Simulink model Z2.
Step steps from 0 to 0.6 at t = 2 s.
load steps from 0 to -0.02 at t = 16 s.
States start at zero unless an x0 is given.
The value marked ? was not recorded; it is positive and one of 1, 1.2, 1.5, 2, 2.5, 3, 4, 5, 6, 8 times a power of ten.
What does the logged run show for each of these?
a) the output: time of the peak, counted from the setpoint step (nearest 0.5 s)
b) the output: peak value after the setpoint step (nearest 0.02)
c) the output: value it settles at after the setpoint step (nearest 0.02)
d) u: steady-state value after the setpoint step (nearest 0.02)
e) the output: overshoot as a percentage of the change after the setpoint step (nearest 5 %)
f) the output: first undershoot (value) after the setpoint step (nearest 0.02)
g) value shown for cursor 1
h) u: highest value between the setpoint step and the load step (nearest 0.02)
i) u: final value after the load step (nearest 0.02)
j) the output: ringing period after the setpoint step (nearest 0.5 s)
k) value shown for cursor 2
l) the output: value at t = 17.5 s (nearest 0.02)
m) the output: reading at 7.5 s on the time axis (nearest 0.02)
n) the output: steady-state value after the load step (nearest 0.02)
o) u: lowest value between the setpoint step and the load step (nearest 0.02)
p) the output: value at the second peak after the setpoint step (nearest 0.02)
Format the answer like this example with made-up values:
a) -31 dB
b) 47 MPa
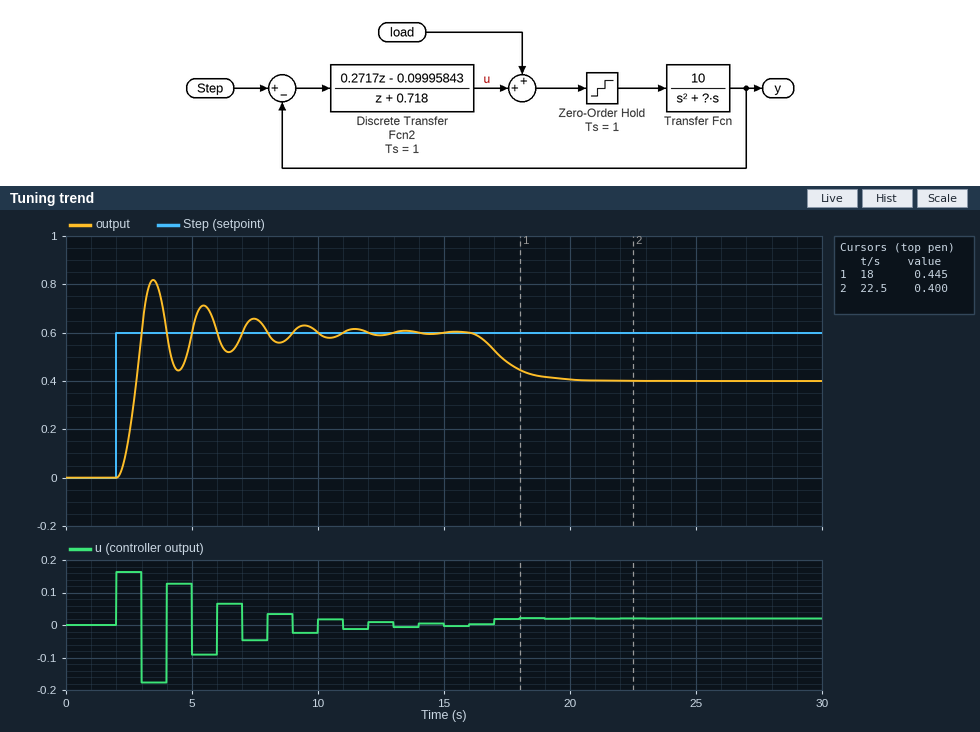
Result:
a) 1.5 s
b) 0.82
c) 0.60
d) 0.00
e) 35 %
f) 0.44
g) 0.445
h) 0.16
i) 0.02
j) 2.0 s
k) 0.400
l) 0.48
m) 0.66
n) 0.40
o) -0.18
p) 0.72
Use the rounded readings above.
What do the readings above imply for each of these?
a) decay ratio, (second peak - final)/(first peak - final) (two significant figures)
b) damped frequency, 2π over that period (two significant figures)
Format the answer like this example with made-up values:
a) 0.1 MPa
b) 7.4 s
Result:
a) 0.55
b) 3.1 rad/s
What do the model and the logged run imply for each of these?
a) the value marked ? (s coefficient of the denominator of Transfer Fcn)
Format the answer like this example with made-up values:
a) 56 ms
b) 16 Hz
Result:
a) 1
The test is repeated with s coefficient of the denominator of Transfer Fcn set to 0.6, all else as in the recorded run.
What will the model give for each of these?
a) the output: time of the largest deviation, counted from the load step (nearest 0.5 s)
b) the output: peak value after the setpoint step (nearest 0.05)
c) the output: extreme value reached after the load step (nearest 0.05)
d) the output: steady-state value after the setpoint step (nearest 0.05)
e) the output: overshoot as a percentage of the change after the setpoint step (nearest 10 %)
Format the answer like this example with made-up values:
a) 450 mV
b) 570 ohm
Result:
a) 3.0 s
b) 1.00
c) 0.40
d) 0.60
e) 60 %
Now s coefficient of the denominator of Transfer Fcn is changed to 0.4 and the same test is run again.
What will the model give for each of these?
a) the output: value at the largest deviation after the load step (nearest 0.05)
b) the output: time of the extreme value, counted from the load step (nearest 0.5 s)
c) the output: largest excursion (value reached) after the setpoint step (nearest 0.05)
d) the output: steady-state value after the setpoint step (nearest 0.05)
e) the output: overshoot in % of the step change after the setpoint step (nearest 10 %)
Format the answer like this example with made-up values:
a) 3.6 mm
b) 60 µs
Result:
a) 0.35
b) 2.5 s
c) 1.10
d) 0.60
e) 80 %
